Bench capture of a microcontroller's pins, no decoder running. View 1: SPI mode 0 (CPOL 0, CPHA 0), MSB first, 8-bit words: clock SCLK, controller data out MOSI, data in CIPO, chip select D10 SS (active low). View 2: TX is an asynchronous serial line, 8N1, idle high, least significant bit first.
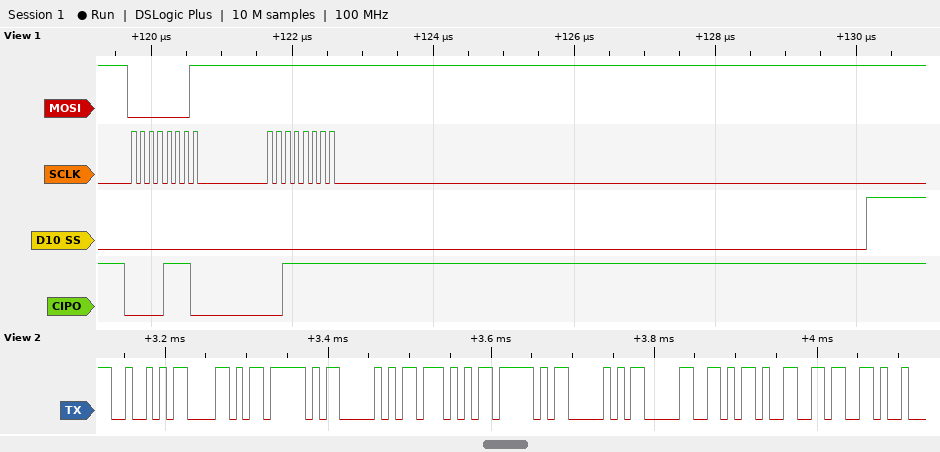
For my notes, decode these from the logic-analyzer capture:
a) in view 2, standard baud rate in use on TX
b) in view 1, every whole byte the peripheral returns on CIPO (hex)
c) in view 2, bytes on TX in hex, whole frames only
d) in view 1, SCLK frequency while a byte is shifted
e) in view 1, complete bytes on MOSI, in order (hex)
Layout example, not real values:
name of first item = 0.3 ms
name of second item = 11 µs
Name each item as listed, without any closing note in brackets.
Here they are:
in view 2, standard baud rate in use on TX = 115200 baud
in view 1, every whole byte the peripheral returns on CIPO = 0E 3F
in view 2, bytes on TX in hex, whole frames only = 0x52 0x58 0x5F 0x50 0x57 0x5F 0x50 0x30 0x2D 0x36
in view 1, SCLK frequency while a byte is shifted = 8 MHz
in view 1, complete bytes on MOSI, in order = 01 FF
